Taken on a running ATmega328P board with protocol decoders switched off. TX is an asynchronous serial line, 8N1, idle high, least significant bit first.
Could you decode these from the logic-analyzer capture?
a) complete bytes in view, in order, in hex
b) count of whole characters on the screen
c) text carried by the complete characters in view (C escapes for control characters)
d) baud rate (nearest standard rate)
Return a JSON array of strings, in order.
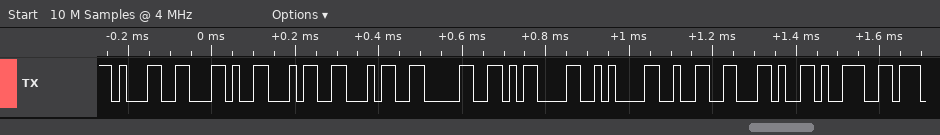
["31 2C 34 34 30 0D 0A 32 2C 39", "10", "\"1,440\\r\\n2,9\"", "57600 baud"]
